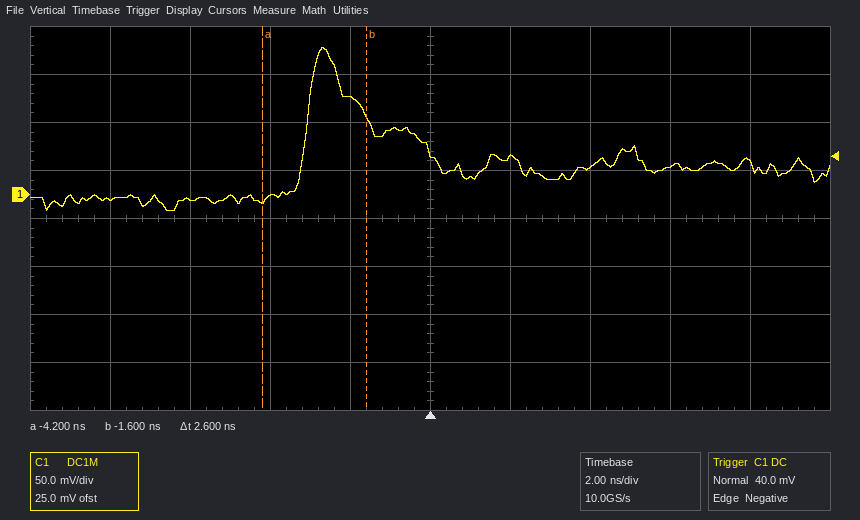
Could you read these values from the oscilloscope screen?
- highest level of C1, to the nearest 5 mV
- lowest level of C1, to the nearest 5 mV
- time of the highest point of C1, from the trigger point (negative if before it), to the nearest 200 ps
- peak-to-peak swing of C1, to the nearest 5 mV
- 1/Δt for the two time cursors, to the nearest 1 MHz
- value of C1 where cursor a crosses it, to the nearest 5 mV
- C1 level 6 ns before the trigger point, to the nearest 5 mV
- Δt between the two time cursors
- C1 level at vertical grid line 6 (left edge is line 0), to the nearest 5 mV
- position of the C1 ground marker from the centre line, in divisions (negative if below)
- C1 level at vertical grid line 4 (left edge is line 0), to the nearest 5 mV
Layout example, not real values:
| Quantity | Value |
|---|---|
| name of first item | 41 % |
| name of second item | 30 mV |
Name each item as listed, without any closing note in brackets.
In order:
| Quantity | Value |
|---|---|
| highest level of C1, to the nearest 5 mV | 155 mV |
| lowest level of C1, to the nearest 5 mV | -15 mV |
| time of the highest point of C1, from the trigger point (negative if before it), to the nearest 200 ps | -2.6 ns |
| peak-to-peak swing of C1, to the nearest 5 mV | 170 mV |
| 1/Δt for the two time cursors, to the nearest 1 MHz | 385 MHz |
| value of C1 where cursor a crosses it, to the nearest 5 mV | -5 mV |
| C1 level 6 ns before the trigger point, to the nearest 5 mV | -5 mV |
| Δt between the two time cursors | 2.6 ns |
| C1 level at vertical grid line 6 (left edge is line 0), to the nearest 5 mV | 40 mV |
| position of the C1 ground marker from the centre line, in divisions | +0.5 div |
| C1 level at vertical grid line 4 (left edge is line 0), to the nearest 5 mV | 100 mV |
